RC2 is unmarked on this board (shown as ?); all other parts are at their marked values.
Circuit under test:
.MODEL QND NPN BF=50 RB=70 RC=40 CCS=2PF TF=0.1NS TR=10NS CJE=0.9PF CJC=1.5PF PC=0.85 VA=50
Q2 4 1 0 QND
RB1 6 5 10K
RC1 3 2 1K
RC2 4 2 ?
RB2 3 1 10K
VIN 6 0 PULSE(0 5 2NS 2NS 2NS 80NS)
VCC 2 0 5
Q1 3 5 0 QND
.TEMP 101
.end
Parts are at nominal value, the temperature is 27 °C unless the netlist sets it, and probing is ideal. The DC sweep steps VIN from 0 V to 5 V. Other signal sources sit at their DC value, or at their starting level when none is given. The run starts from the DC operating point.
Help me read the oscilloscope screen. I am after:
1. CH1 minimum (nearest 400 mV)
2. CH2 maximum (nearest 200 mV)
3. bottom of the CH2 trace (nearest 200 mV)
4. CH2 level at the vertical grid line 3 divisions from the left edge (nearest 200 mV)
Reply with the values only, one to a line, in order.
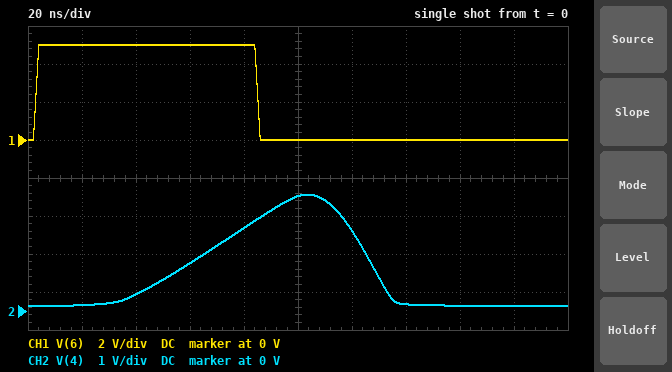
0 V
3.0 V
200 mV
1.2 V
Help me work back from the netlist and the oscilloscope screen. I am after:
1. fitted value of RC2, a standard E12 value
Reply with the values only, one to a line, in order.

2.7 kΩ
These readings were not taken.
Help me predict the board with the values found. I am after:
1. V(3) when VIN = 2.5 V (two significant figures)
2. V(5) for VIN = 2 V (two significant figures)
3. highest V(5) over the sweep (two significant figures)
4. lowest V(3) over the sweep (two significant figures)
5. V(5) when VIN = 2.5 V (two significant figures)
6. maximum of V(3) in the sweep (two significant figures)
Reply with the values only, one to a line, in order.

320 mV
730 mV
750 mV
280 mV
730 mV
4.6 V
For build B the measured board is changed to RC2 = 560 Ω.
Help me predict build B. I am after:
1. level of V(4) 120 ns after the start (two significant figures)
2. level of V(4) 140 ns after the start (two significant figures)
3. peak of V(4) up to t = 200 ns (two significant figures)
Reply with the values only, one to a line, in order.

4.1 V
1.7 V
5.0 V
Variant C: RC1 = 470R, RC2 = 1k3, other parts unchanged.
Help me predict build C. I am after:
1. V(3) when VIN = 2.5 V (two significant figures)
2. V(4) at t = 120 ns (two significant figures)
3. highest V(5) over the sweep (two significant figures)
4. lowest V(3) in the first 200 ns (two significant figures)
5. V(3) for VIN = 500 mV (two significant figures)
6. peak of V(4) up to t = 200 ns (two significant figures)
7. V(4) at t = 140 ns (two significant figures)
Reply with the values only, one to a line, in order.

900 mV
870 mV
770 mV
510 mV
4.8 V
3.0 V
240 mV
